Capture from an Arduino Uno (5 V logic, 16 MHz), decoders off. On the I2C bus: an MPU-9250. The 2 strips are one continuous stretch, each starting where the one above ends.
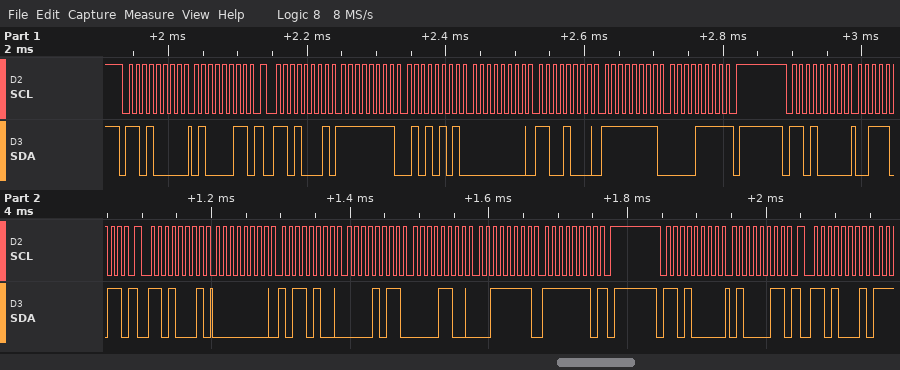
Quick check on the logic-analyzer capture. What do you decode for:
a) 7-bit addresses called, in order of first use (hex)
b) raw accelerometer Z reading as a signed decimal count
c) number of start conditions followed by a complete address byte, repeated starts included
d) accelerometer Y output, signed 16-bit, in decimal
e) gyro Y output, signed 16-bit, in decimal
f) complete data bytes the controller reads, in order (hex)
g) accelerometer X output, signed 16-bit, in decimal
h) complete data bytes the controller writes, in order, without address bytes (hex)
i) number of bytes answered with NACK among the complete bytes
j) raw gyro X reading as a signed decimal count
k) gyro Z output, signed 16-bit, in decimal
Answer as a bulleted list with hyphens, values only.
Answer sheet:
- 0x68
- 16382
- 6
- 2828
- 200
- FF 55 00 C8 FF 0F 00 B4 0B 0C 3F FE
- 180
- 43 3B 43
- 2
- -171
- -241
